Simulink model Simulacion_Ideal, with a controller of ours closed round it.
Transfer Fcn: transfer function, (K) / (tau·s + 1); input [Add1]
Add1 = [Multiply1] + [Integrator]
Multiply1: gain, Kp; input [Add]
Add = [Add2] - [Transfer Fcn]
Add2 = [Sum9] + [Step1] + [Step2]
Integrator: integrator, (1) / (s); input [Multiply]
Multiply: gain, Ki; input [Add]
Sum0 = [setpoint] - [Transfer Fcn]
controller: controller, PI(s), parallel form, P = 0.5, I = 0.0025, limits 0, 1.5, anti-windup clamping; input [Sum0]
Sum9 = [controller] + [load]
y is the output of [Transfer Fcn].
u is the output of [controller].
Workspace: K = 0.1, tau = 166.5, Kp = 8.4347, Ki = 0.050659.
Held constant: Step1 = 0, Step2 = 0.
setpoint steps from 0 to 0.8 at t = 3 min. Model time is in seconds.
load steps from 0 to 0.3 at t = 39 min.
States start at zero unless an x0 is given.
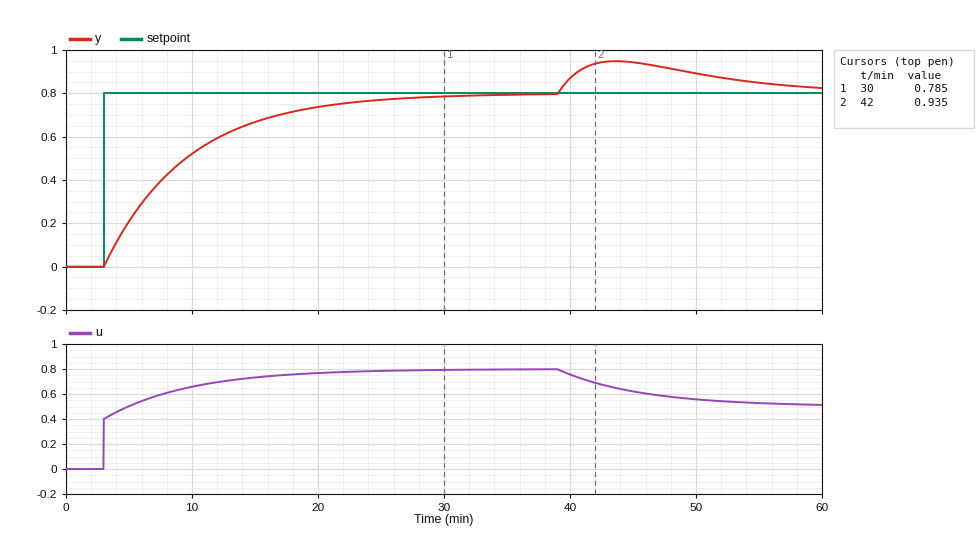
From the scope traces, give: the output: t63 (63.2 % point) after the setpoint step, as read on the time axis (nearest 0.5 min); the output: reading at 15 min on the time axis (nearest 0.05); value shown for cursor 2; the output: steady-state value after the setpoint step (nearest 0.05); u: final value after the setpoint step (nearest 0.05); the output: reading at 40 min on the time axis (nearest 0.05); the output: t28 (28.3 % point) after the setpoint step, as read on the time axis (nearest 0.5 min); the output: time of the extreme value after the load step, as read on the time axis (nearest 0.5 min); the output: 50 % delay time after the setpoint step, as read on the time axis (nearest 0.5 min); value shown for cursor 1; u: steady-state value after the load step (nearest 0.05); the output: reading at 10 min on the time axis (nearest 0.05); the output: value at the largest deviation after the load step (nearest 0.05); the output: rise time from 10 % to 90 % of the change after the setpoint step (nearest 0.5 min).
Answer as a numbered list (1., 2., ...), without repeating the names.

1. 9.5 min
2. 0.65
3. 0.935
4. 0.80
5. 0.80
6. 0.85
7. 5.0 min
8. 43.5 min
9. 7.5 min
10. 0.785
11. 0.50
12. 0.50
13. 0.95
14. 14.5 min
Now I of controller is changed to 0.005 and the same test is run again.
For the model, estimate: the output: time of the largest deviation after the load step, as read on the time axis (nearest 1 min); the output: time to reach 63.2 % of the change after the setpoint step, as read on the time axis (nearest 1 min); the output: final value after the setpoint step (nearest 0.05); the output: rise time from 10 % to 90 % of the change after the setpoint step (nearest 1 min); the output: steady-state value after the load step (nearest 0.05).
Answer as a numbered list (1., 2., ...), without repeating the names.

1. 43 min
2. 7 min
3. 0.80
4. 7 min
5. 0.80
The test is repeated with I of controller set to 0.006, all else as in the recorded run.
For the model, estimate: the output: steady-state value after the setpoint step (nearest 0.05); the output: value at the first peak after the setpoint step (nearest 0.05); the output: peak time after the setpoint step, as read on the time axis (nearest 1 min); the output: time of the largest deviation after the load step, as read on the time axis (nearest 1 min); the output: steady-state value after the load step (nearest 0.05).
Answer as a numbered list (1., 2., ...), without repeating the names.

1. 0.80
2. 0.85
3. 14 min
4. 42 min
5. 0.80
